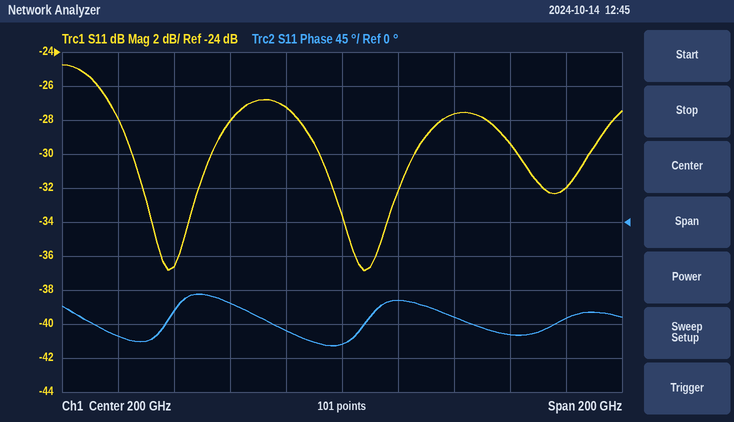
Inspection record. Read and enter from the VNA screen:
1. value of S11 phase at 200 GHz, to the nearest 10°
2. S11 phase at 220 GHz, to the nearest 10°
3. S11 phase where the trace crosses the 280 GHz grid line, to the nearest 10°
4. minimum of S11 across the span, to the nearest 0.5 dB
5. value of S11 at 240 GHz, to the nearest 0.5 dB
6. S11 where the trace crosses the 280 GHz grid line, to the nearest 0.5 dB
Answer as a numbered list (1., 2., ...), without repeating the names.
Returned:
1. -160°
2. -100°
3. -130°
4. -37.0 dB
5. -27.5 dB
6. -32.0 dB
